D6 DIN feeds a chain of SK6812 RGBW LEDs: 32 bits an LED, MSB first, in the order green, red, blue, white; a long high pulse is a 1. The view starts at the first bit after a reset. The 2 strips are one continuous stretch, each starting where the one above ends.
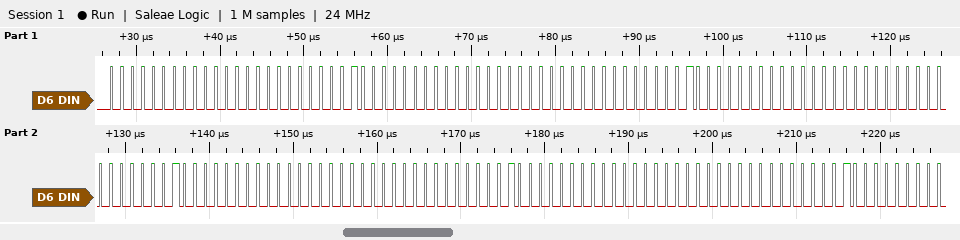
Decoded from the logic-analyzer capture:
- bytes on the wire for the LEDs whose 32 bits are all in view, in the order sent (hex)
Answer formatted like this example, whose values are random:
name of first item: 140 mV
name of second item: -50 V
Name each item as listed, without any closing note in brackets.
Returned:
bytes on the wire for the LEDs whose 32 bits are all in view, in the order sent: 00 00 01 00 00 00 01 00 00 00 01 00 00 00 01 00 00 00 01 00
